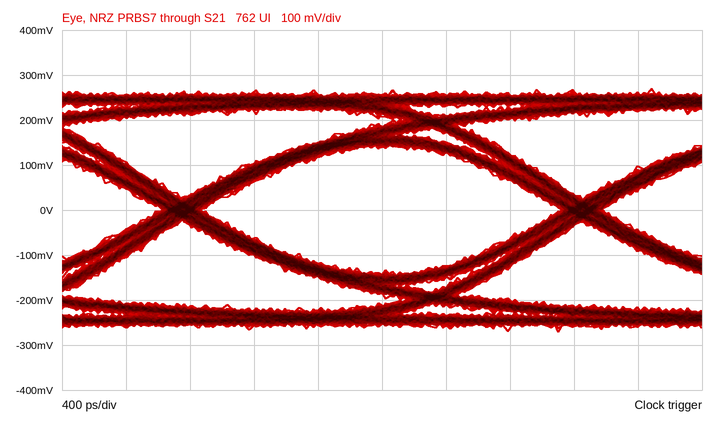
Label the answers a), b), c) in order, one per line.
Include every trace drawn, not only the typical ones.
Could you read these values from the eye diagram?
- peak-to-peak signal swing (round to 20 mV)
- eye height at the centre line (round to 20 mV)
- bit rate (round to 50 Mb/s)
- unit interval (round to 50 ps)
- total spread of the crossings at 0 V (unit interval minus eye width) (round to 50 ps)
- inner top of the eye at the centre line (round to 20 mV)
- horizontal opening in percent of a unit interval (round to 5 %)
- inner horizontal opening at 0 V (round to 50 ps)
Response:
a) 540 mV
b) 280 mV
c) 400 Mb/s
d) 2.50 ns
e) 250 ps
f) 140 mV
g) 90 %
h) 2.25 ns
